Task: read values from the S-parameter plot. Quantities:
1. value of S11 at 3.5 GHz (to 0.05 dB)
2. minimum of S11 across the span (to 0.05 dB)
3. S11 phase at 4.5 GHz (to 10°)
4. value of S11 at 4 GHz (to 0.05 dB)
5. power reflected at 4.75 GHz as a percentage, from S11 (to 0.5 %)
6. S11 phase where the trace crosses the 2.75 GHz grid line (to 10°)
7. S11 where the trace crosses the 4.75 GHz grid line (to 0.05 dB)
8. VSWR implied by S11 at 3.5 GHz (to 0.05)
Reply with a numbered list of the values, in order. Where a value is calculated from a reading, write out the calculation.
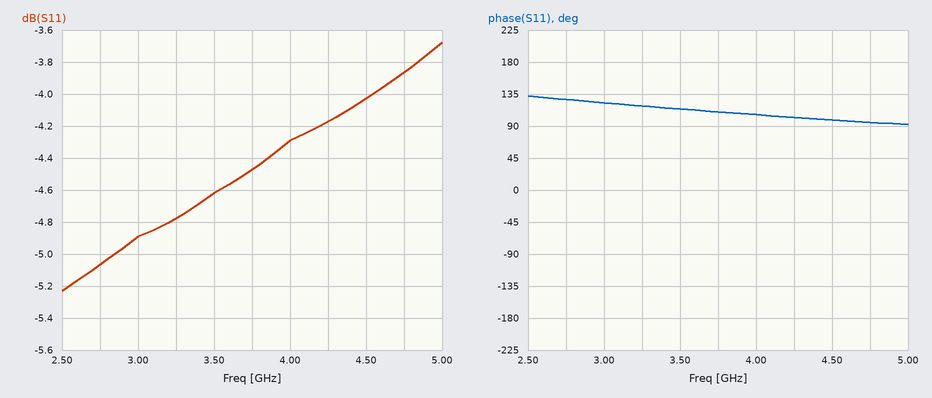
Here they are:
1. -4.60 dB
2. -5.25 dB
3. 100°
4. -4.30 dB
5. 10^(-3.85/10) ≈ 41.2 %, so 41.0 % to the nearest 0.5 %
6. 130°
7. -3.85 dB
8. |Γ| = 10^(-4.6/20) = 0.5888; VSWR = (1 + 0.5888)/(1 − 0.5888) ≈ 3.86, so 3.85 to the nearest 0.05
